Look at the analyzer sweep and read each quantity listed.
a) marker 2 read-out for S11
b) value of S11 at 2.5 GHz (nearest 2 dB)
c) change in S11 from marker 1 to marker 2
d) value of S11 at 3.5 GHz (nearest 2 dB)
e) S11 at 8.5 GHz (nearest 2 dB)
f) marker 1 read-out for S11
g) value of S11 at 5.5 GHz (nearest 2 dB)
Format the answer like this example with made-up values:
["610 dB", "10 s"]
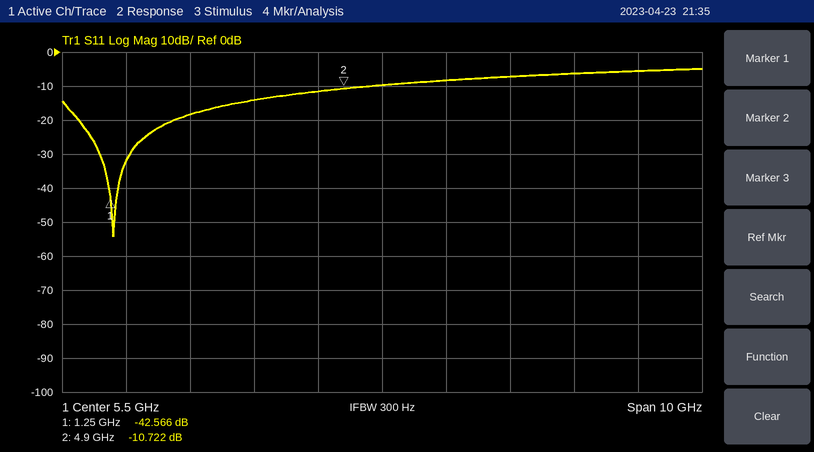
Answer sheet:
["-10.722 dB", "-18 dB", "31.844 dB", "-14 dB", "-6 dB", "-42.566 dB", "-10 dB"]
